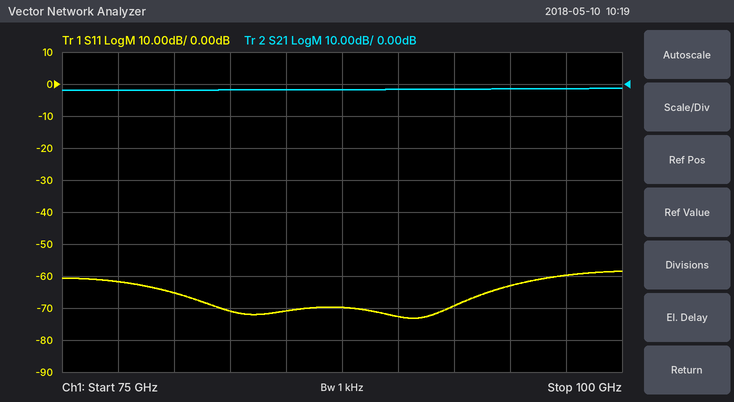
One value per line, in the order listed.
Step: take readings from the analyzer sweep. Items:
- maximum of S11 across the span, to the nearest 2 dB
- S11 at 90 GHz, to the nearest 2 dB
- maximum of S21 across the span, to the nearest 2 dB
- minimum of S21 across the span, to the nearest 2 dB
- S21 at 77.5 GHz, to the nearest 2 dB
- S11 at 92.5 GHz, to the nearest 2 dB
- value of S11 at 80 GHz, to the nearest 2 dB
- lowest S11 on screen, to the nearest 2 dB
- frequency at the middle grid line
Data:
-58 dB
-72 dB
-2 dB
-2 dB
-2 dB
-70 dB
-66 dB
-74 dB
87.5 GHz
